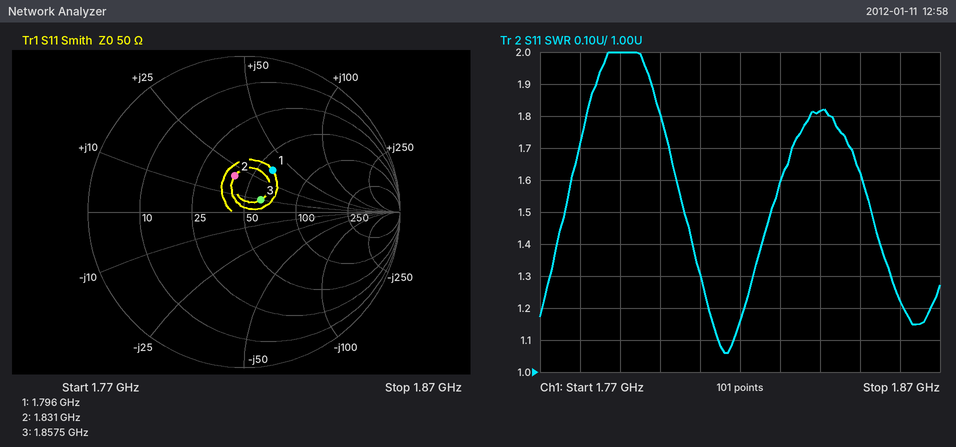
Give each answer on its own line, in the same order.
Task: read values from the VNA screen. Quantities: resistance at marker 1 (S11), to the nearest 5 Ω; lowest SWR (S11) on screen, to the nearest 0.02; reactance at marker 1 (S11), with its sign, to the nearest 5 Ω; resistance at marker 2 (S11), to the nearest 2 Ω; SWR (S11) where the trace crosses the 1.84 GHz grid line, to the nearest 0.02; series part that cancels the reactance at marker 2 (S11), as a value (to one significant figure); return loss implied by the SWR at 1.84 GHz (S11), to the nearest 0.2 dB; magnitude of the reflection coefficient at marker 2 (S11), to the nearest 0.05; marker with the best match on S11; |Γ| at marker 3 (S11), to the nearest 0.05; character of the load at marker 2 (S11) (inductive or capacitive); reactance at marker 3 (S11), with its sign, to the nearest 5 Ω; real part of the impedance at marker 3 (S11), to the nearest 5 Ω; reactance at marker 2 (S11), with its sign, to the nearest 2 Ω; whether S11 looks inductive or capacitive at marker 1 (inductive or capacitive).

60 Ω
1.06
+35 Ω
40 Ω
1.82
4 pF
10.8 dB
0.25
marker 3
0.15
inductive
+10 Ω
60 Ω
+20 Ω
inductive
